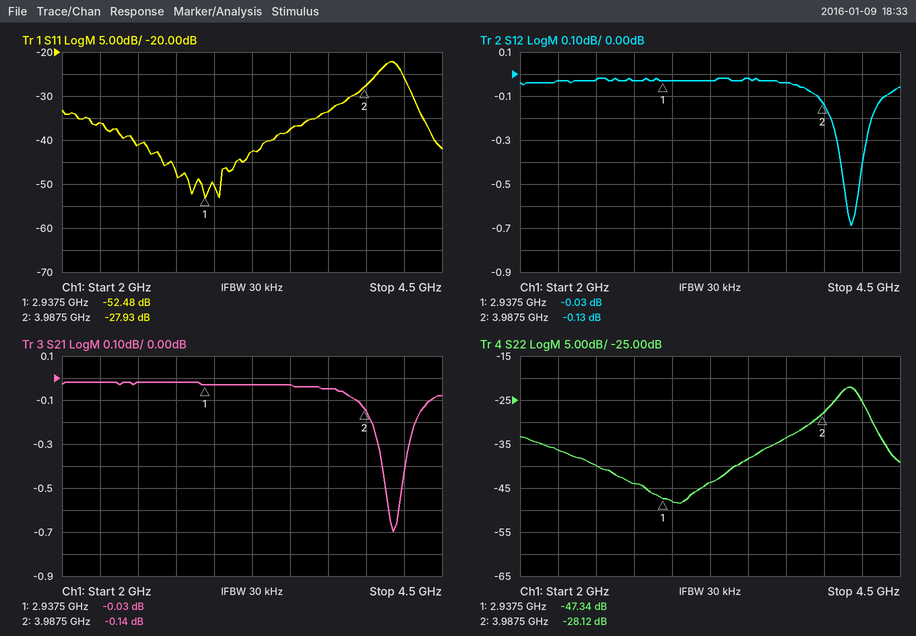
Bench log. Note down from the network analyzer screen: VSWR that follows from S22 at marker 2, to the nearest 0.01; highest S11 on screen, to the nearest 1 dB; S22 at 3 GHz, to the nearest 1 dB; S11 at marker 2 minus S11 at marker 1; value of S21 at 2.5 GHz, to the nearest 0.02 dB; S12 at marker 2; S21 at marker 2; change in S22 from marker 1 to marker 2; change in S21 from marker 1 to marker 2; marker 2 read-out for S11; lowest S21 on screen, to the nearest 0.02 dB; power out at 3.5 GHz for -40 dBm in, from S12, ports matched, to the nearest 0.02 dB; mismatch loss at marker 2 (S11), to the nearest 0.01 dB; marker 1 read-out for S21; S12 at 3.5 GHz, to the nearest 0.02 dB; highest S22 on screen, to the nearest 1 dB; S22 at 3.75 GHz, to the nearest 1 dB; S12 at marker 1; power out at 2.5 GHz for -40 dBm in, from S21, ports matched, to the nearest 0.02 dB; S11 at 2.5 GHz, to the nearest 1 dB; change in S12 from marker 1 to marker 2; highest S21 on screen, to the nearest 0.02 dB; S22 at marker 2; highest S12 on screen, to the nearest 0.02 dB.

1.08
-22 dB
-48 dB
24.55 dB
-0.02 dB
-0.13 dB
-0.14 dB
19.22 dB
-0.11 dB
-27.93 dB
-0.70 dB
-40.02 dBm
0.01 dB
-0.03 dB
-0.02 dB
-22 dB
-34 dB
-0.03 dB
-40.02 dBm
-41 dB
-0.10 dB
-0.02 dB
-28.12 dB
-0.02 dB
